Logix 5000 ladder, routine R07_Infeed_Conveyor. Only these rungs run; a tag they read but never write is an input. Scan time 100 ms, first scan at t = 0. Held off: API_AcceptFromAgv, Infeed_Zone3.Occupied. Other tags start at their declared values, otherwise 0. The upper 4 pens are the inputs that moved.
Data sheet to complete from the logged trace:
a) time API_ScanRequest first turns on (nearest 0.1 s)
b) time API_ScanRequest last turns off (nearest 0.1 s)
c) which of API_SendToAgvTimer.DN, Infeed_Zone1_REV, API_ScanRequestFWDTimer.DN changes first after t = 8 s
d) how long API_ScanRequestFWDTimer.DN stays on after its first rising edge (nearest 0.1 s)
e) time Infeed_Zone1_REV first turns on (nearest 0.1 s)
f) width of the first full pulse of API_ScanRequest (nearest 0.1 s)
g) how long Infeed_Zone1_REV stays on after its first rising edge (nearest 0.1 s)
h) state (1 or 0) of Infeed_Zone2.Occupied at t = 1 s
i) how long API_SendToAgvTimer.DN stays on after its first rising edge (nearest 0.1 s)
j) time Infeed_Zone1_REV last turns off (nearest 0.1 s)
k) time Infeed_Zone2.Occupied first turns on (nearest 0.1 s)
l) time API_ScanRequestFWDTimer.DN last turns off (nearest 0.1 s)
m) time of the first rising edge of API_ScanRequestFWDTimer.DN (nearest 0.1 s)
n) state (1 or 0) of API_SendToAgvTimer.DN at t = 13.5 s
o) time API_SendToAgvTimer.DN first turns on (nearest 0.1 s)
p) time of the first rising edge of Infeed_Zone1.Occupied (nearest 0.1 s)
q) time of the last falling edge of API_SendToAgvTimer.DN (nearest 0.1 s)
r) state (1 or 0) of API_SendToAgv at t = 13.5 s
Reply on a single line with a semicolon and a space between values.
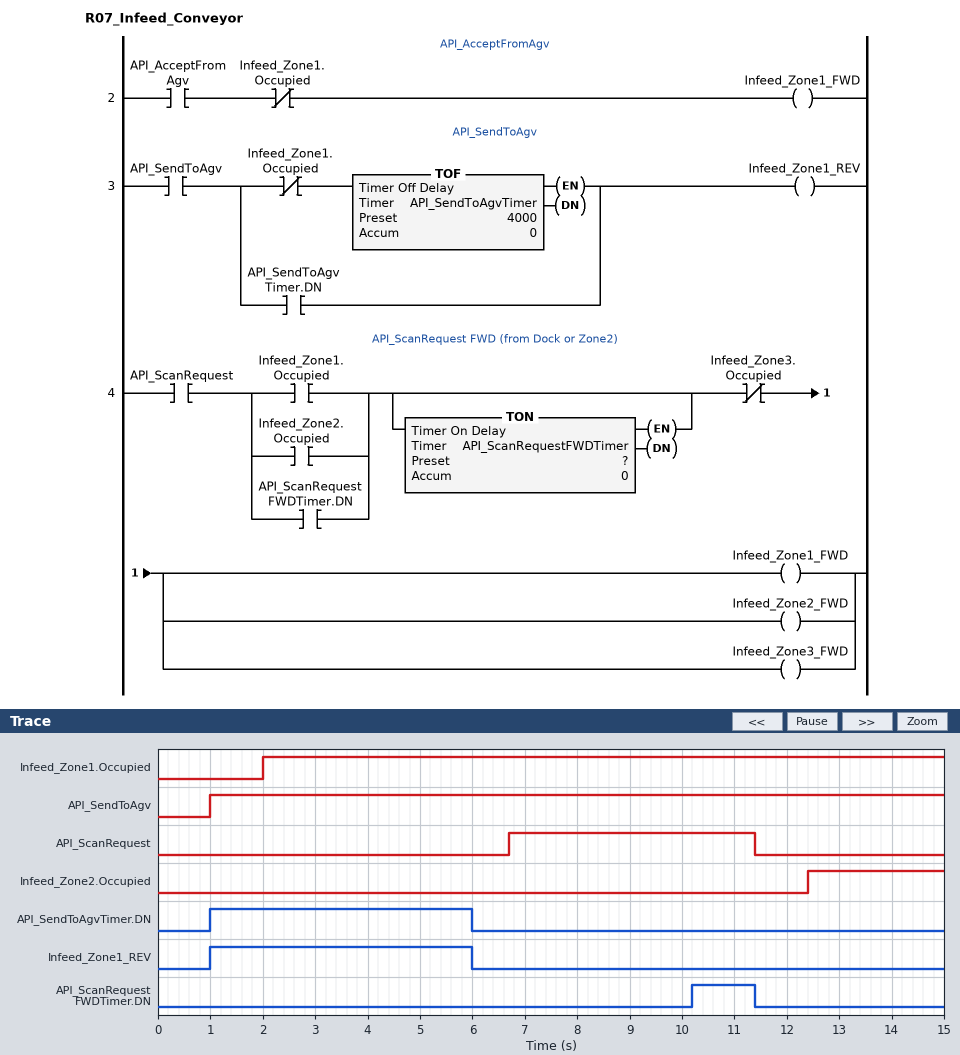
6.7 s; 11.4 s; API_ScanRequestFWDTimer.DN; 1.2 s; 1.0 s; 4.7 s; 5.0 s; 0; 5.0 s; 6.0 s; 12.4 s; 11.4 s; 10.2 s; 0; 1.0 s; 2.0 s; 6.0 s; 1
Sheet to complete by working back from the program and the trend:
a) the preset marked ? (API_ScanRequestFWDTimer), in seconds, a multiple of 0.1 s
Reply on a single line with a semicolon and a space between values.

3.5 s
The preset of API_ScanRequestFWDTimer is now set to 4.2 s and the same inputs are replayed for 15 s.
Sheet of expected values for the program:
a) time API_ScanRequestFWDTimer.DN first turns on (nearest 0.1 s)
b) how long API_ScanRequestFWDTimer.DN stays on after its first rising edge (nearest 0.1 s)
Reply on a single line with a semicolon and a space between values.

10.9 s; 0.5 s
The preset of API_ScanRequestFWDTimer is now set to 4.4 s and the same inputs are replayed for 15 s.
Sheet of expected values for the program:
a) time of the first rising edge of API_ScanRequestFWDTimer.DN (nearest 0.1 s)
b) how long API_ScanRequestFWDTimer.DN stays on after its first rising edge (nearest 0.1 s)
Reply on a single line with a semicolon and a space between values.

11.1 s; 0.3 s
